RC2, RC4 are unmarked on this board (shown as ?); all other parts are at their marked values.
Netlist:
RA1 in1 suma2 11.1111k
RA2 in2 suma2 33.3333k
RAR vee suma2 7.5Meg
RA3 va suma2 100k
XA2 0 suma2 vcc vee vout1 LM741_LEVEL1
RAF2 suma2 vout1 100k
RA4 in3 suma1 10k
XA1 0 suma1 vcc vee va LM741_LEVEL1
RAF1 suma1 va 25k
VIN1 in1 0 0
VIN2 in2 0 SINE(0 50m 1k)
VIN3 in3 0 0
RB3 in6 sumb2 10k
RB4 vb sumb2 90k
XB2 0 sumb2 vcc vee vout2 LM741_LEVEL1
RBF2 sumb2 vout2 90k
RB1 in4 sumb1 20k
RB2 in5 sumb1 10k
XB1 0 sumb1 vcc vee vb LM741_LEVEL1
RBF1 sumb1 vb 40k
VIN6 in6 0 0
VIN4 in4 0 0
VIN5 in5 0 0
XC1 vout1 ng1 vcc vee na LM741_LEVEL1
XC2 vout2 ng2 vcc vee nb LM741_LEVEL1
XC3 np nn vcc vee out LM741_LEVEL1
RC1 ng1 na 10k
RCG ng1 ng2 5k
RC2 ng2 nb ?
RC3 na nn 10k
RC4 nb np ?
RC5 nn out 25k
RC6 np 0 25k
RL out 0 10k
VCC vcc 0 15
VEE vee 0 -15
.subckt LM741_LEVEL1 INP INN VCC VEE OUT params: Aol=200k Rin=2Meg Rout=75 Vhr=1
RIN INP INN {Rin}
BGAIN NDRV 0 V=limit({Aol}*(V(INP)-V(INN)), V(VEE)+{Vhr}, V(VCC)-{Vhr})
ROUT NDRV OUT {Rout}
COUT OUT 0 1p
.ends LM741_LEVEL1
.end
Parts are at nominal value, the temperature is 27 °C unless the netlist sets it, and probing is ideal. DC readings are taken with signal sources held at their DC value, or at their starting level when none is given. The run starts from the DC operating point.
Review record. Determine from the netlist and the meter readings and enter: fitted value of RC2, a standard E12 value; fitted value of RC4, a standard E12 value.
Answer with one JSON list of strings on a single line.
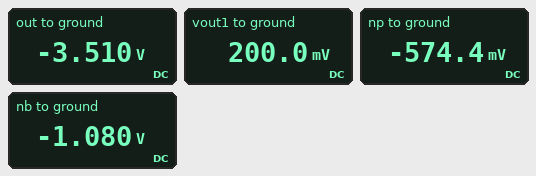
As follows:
["27 kΩ", "22 kΩ"]
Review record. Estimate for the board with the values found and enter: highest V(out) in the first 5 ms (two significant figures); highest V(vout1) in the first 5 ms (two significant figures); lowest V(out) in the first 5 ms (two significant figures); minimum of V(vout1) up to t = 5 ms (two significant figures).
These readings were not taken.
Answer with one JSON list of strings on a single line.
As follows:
["-880 mV", "350 mV", "-6.1 V", "50 mV"]
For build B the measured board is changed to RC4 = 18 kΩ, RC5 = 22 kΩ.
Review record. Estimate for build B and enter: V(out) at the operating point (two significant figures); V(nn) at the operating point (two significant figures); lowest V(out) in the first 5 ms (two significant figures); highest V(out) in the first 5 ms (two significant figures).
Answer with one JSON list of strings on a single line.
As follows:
["-3.3 V", "-630 mV", "-5.8 V", "-830 mV"]
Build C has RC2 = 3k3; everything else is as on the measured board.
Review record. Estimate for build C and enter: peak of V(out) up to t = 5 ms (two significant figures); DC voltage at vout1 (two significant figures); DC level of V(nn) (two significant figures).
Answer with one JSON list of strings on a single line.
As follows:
["-440 mV", "200 mV", "-70 mV"]
